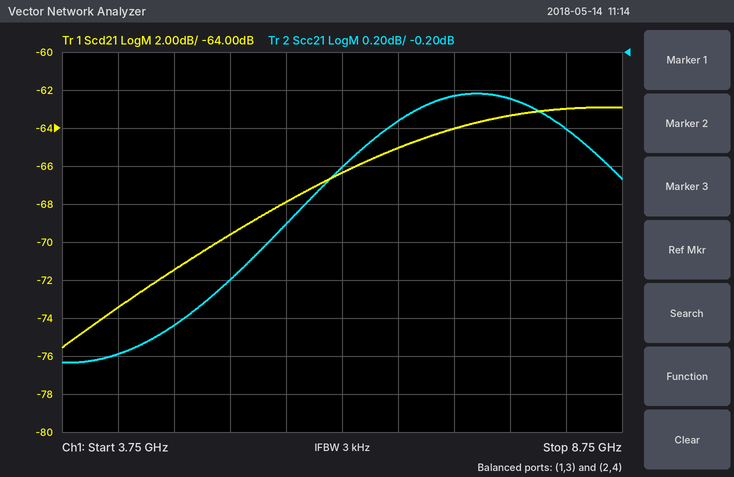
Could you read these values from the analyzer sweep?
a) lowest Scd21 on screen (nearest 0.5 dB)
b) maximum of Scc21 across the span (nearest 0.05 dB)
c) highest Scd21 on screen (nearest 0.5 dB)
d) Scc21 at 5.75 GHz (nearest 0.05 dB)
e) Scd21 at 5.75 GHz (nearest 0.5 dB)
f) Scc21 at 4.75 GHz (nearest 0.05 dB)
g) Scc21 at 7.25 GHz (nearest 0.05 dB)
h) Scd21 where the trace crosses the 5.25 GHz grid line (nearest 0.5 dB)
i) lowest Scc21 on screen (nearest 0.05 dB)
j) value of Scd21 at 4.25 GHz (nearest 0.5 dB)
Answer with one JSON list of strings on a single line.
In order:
["-75.5 dB", "-0.40 dB", "-63.0 dB", "-1.10 dB", "-68.0 dB", "-1.65 dB", "-0.45 dB", "-69.5 dB", "-1.85 dB", "-73.5 dB"]
